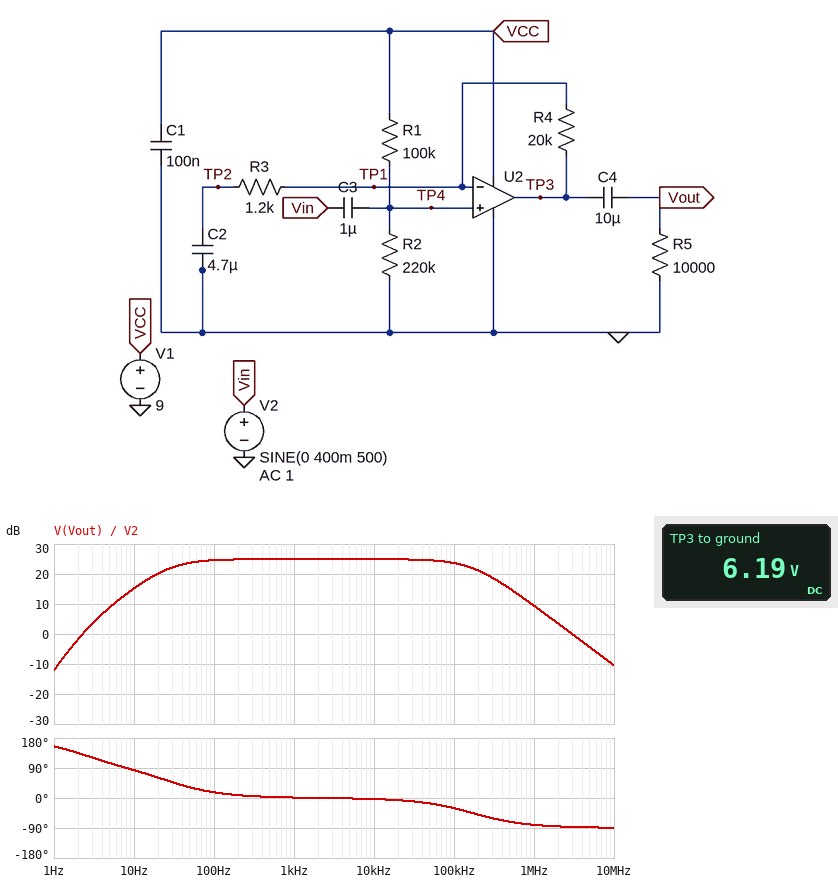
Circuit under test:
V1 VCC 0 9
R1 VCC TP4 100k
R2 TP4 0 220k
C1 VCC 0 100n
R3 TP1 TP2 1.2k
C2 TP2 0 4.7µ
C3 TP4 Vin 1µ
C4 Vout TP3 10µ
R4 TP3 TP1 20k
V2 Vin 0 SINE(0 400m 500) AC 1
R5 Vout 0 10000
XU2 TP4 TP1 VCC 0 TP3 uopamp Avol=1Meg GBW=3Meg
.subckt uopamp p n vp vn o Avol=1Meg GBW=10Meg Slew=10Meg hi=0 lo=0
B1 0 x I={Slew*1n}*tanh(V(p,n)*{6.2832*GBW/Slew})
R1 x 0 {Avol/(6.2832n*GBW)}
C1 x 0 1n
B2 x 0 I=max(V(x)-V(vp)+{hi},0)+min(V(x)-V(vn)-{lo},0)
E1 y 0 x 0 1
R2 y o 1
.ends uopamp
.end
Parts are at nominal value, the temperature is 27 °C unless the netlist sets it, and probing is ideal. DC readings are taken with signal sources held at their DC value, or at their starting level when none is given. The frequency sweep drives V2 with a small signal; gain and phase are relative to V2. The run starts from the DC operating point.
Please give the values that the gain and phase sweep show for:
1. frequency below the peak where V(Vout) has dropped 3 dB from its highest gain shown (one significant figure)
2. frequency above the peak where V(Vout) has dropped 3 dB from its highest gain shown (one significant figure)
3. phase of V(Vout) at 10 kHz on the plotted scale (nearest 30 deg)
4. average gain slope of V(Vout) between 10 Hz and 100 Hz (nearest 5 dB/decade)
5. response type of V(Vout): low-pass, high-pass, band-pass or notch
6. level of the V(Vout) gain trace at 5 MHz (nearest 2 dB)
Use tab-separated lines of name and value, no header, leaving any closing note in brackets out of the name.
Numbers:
frequency below the peak where V(Vout) has dropped 3 dB from its highest gain shown	30 Hz
frequency above the peak where V(Vout) has dropped 3 dB from its highest gain shown	200 kHz
phase of V(Vout) at 10 kHz on the plotted scale	0 deg
average gain slope of V(Vout) between 10 Hz and 100 Hz	10 dB/decade
response type of V(Vout): low-pass, high-pass, band-pass or notch	band-pass
level of the V(Vout) gain trace at 5 MHz	-4 dB
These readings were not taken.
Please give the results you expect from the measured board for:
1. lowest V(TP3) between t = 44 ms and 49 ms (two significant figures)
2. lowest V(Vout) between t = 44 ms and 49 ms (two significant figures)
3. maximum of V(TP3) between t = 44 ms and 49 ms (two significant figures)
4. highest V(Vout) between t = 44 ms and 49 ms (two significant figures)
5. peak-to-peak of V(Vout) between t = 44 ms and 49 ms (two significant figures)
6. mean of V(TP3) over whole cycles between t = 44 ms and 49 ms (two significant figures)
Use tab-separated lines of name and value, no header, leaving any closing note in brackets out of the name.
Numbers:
lowest V(TP3) between t = 44 ms and 49 ms	670 mV
lowest V(Vout) between t = 44 ms and 49 ms	-5.4 V
maximum of V(TP3) between t = 44 ms and 49 ms	9.0 V
highest V(Vout) between t = 44 ms and 49 ms	2.9 V
peak-to-peak of V(Vout) between t = 44 ms and 49 ms	8.3 V
mean of V(TP3) over whole cycles between t = 44 ms and 49 ms	6.1 V
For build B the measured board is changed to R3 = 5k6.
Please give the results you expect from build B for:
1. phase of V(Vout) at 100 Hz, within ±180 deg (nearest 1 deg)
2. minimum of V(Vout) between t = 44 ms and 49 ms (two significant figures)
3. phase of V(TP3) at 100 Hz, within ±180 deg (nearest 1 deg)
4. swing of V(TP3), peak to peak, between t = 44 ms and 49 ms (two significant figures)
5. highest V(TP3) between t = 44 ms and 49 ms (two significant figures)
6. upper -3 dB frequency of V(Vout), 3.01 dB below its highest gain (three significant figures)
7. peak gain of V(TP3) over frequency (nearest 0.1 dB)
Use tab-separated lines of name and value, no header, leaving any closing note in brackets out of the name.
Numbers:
phase of V(Vout) at 100 Hz, within ±180 deg	5 deg
minimum of V(Vout) between t = 44 ms and 49 ms	-1.8 V
phase of V(TP3) at 100 Hz, within ±180 deg	4 deg
swing of V(TP3), peak to peak, between t = 44 ms and 49 ms	3.7 V
highest V(TP3) between t = 44 ms and 49 ms	8.0 V
upper -3 dB frequency of V(Vout), 3.01 dB below its highest gain	656 kHz
peak gain of V(TP3) over frequency	13.2 dB
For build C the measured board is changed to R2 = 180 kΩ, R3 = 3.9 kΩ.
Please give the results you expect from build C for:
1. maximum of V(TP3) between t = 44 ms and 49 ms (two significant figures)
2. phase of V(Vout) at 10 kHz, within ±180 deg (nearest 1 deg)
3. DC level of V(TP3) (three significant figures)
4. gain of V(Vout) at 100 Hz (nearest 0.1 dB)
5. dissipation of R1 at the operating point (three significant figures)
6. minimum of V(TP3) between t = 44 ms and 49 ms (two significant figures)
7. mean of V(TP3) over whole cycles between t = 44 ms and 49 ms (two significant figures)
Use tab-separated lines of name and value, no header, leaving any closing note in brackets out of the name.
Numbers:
maximum of V(TP3) between t = 44 ms and 49 ms	8.2 V
phase of V(Vout) at 10 kHz, within ±180 deg	-1 deg
DC level of V(TP3)	5.79 V
gain of V(Vout) at 100 Hz	15.7 dB
dissipation of R1 at the operating point	103 µW
minimum of V(TP3) between t = 44 ms and 49 ms	3.3 V
mean of V(TP3) over whole cycles between t = 44 ms and 49 ms	5.8 V
